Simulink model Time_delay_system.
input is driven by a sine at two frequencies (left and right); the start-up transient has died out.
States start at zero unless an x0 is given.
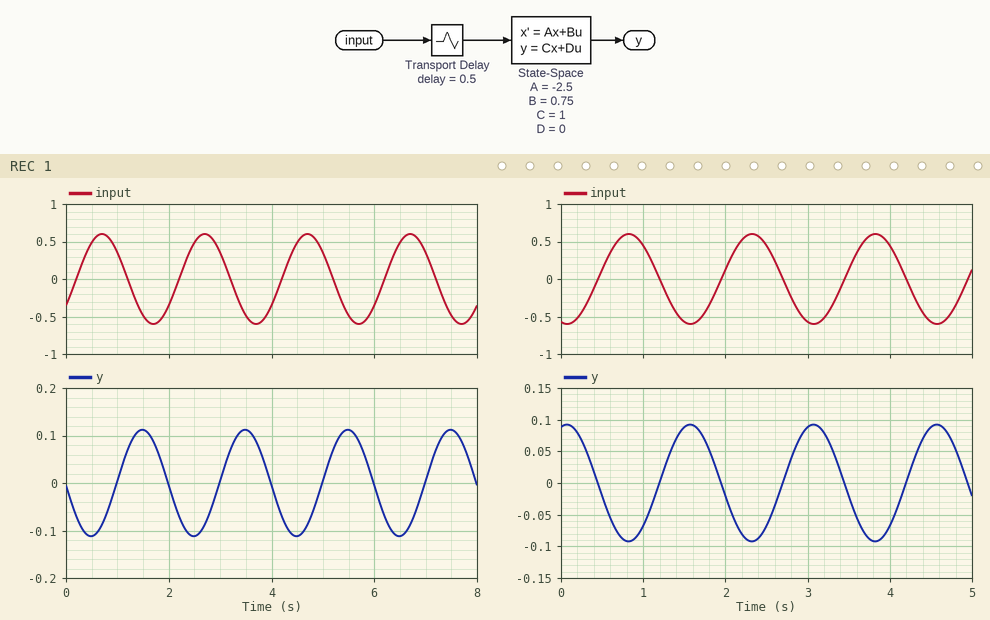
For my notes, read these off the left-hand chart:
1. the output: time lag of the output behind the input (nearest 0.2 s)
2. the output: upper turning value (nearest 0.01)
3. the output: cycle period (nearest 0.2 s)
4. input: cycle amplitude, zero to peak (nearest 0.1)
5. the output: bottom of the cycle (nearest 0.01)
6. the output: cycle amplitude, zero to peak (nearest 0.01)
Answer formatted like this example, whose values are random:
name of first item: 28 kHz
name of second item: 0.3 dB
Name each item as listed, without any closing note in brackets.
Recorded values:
the output: time lag of the output behind the input: 0.8 s
the output: upper turning value: 0.11
the output: cycle period: 2.0 s
input: cycle amplitude, zero to peak: 0.6
the output: bottom of the cycle: -0.11
the output: cycle amplitude, zero to peak: 0.11
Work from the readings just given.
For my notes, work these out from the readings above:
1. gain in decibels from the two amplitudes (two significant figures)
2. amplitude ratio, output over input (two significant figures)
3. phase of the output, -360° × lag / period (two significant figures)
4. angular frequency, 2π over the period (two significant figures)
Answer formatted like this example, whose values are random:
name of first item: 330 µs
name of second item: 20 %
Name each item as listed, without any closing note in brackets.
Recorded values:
gain in decibels from the two amplitudes: -15 dB
amplitude ratio, output over input: 0.18
phase of the output, -360° × lag / period: -140°
angular frequency, 2π over the period: 3.1 rad/s
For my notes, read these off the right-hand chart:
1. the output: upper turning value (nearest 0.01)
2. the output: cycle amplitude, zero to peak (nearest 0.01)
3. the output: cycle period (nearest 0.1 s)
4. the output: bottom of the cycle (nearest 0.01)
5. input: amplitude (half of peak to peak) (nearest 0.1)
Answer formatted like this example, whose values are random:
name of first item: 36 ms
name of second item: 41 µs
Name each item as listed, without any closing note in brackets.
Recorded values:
the output: upper turning value: 0.09
the output: cycle amplitude, zero to peak: 0.09
the output: cycle period: 1.5 s
the output: bottom of the cycle: -0.09
input: amplitude (half of peak to peak): 0.6
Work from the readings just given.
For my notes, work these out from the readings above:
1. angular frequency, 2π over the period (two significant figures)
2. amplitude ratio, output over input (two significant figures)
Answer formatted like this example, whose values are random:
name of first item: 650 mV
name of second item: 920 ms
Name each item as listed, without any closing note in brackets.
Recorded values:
angular frequency, 2π over the period: 4.2 rad/s
amplitude ratio, output over input: 0.15
